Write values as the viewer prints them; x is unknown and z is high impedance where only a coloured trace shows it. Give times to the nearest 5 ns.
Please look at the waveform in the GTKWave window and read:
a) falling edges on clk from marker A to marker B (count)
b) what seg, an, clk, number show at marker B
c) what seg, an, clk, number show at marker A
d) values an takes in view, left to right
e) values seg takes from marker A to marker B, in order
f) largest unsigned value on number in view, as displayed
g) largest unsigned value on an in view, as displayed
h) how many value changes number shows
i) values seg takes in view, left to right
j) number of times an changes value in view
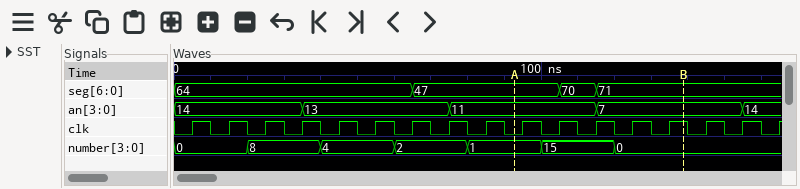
4
seg=71, an=7, clk=1, number=0
seg=47, an=11, clk=0, number=1
14, 13, 11, 7, 14
47, 70, 71
15
14
6
64, 47, 70, 71
4
